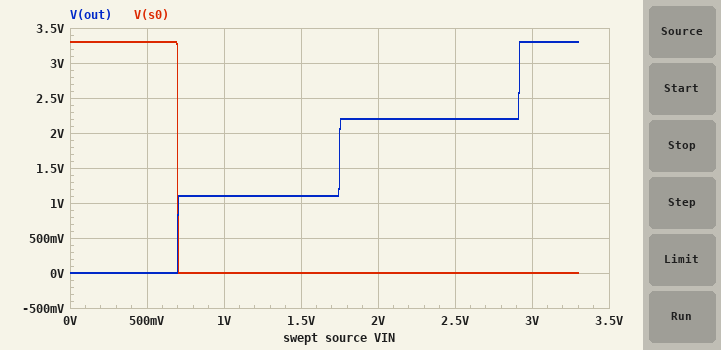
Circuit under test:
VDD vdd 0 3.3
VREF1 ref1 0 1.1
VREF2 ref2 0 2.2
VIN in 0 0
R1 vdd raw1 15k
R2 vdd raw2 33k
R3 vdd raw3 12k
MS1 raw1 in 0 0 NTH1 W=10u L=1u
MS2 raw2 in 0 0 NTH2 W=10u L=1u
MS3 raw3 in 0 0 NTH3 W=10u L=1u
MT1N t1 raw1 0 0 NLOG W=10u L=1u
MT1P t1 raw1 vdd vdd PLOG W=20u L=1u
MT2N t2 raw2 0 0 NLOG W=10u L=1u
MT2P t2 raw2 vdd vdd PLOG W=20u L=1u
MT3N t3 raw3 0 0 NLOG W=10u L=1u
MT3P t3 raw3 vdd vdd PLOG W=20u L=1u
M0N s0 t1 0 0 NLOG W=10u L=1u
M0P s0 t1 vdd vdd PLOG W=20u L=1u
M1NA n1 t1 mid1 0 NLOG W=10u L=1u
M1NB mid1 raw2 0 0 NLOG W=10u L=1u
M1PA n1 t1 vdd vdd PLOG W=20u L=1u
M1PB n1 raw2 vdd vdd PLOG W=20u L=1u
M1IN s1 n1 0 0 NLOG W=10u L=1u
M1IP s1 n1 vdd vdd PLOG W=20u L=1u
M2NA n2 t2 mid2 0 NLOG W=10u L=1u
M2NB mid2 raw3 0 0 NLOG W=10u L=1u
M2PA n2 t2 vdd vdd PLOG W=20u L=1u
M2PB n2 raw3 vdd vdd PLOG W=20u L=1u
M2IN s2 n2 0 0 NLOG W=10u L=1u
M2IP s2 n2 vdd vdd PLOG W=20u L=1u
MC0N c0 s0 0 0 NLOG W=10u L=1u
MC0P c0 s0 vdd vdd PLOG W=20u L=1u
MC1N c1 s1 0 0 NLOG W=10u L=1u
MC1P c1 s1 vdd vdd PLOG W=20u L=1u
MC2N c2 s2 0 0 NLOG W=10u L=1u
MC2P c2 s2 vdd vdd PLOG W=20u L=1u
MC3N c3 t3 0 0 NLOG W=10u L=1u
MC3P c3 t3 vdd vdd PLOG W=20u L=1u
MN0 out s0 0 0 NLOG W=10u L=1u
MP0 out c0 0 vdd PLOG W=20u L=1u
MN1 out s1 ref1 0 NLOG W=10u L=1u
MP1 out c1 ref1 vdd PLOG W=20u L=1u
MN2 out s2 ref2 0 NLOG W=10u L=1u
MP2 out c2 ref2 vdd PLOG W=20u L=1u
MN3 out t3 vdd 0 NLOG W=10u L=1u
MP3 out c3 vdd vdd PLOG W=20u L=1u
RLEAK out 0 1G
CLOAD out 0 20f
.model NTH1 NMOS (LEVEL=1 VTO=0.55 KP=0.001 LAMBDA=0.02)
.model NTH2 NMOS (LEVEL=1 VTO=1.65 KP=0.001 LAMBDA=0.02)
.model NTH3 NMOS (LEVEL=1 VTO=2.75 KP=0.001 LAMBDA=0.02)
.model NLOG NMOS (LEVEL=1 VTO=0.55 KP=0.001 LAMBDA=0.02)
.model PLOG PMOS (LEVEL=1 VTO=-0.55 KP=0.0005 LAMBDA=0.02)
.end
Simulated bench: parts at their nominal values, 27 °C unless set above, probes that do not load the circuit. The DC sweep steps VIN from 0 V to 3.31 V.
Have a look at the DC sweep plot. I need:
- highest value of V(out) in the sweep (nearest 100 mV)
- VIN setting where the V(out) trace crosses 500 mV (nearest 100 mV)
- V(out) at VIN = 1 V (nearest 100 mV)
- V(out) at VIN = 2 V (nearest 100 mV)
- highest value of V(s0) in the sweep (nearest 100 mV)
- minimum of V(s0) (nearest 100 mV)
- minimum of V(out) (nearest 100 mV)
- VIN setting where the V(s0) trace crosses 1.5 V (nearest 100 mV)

3.3 V
700 mV
1.1 V
2.2 V
3.3 V
0 V
0 V
700 mV
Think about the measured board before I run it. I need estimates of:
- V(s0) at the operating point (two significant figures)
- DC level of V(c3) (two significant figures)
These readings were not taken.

3.3 V
3.3 V
